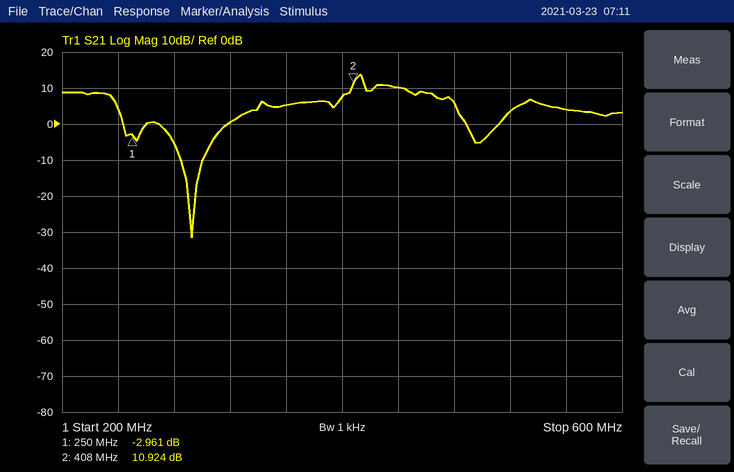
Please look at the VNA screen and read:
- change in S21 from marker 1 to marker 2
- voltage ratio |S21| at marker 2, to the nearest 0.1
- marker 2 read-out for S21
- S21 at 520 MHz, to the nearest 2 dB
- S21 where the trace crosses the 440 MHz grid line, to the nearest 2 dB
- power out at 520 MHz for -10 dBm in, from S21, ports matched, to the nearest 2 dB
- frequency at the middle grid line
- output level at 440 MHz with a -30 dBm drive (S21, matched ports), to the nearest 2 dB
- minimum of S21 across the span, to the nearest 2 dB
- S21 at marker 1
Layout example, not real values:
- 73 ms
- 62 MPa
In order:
- 13.885 dB
- 3.5
- 10.924 dB
- 4 dB
- 10 dB
- -6 dBm
- 400 MHz
- -20 dBm
- -32 dB
- -2.961 dB
